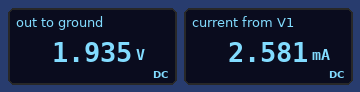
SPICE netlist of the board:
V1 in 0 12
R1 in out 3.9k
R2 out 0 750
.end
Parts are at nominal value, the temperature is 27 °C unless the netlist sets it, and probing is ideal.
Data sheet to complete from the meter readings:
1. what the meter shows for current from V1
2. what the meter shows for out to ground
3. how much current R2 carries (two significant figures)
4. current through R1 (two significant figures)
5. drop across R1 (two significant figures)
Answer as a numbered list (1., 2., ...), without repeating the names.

1. 2.581 mA
2. 1.935 V
3. 2.6 mA
4. 2.6 mA
5. 10 V
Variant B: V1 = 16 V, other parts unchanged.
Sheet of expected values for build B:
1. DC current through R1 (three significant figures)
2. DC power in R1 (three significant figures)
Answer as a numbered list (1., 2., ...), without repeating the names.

1. 3.44 mA
2. 46.2 mW
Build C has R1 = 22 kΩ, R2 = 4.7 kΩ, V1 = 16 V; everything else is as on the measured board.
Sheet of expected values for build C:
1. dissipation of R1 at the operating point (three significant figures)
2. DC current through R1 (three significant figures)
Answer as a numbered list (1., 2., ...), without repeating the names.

1. 7.90 mW
2. 599 µA
